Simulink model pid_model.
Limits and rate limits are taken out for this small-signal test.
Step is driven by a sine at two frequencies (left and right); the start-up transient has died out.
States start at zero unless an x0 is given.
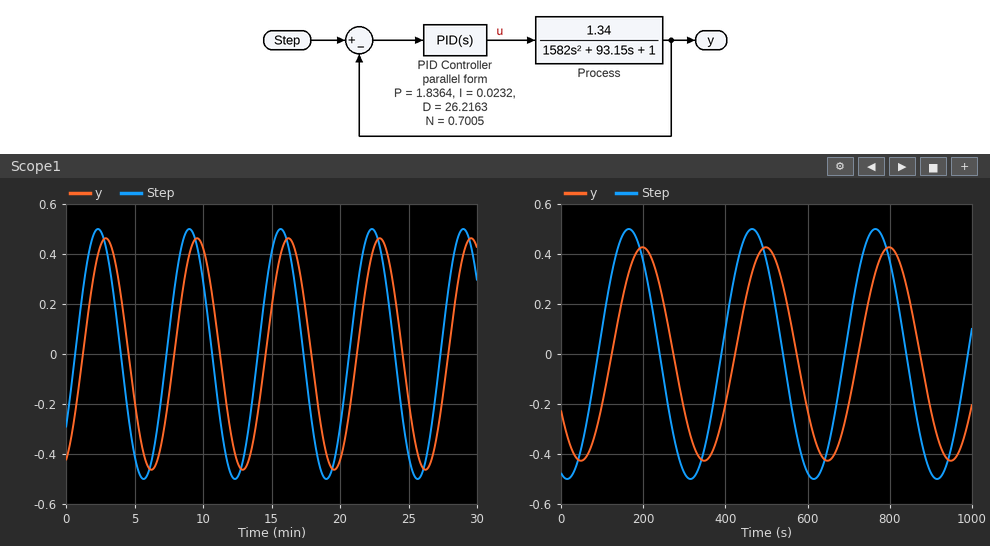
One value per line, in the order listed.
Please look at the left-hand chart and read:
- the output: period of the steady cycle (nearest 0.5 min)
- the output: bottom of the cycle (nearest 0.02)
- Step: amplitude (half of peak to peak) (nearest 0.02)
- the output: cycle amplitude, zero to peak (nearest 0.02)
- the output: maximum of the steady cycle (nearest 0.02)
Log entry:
6.5 min
-0.46
0.50
0.46
0.46
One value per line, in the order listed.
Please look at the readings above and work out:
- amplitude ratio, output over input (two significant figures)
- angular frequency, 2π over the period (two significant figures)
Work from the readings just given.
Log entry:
0.92
0.97 rad/min
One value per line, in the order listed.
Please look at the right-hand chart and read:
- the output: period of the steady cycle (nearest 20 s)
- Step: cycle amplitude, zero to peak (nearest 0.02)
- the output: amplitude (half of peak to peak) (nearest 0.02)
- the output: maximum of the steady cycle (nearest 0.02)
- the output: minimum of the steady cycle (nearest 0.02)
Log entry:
300 s
0.50
0.42
0.42
-0.42
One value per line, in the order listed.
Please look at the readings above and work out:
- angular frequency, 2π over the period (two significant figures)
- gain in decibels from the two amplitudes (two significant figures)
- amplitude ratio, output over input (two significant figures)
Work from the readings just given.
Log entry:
0.021 rad/s
-1.5 dB
0.84
